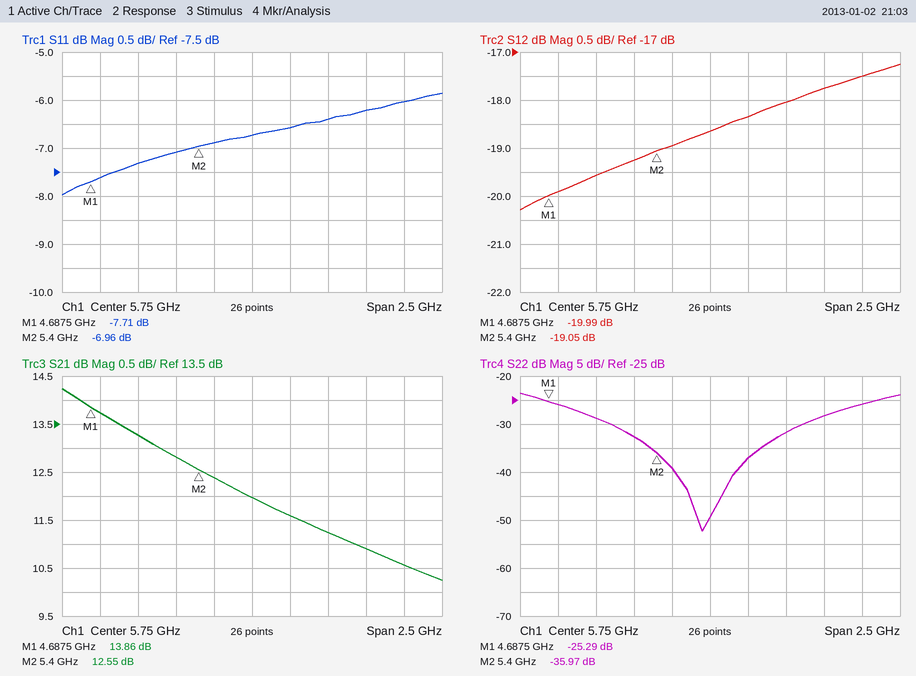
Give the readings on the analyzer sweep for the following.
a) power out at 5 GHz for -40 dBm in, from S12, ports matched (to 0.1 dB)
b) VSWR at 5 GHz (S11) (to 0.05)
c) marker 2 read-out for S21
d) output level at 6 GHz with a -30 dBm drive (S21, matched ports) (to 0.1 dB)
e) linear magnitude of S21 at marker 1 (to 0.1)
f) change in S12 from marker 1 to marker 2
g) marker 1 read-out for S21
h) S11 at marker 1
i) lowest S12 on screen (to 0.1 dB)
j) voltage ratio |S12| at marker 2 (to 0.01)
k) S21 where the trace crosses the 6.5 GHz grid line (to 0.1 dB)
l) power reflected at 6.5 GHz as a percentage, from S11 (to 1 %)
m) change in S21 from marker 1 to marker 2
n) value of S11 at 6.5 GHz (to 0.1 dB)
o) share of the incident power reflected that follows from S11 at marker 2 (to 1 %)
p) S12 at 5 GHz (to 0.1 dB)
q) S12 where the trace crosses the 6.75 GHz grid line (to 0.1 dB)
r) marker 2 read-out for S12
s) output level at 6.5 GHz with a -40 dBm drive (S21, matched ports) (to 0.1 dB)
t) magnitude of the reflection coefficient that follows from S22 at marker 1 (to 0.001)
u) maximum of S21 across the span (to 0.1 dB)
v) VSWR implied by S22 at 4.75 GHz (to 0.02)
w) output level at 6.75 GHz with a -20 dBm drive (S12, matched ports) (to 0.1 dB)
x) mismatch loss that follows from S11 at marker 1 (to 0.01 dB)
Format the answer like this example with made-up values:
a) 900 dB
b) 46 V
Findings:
a) -59.6 dBm
b) 2.50
c) 12.55 dB
d) -18.4 dBm
e) 4.9
f) 0.94 dB
g) 13.86 dB
h) -7.71 dB
i) -20.3 dB
j) 0.11
k) 10.9 dB
l) 24 %
m) -1.31 dB
n) -6.2 dB
o) 20 %
p) -19.6 dB
q) -17.5 dB
r) -19.05 dB
s) -29.1 dBm
t) 0.054
u) 14.2 dB
v) 1.10
w) -37.5 dBm
x) 0.81 dB
